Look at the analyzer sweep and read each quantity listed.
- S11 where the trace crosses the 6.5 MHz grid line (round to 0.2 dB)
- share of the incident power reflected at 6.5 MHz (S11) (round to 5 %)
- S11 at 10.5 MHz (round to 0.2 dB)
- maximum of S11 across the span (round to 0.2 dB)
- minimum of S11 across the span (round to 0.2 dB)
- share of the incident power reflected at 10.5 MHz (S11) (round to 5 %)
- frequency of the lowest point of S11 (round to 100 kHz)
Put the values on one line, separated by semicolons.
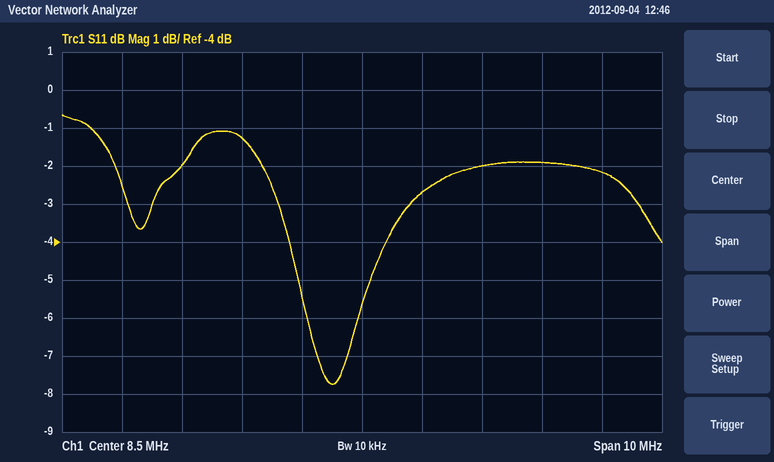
-1.2 dB; 75 %; -2.0 dB; -0.6 dB; -7.8 dB; 65 %; 8.0 MHz
